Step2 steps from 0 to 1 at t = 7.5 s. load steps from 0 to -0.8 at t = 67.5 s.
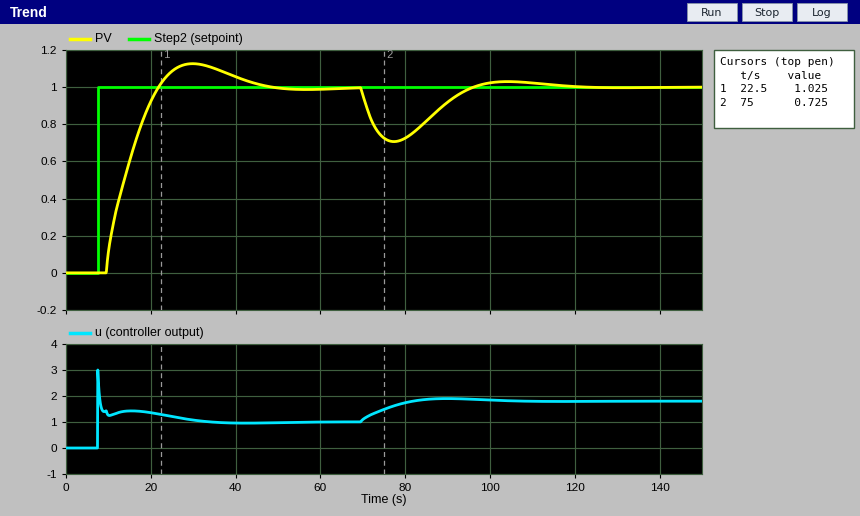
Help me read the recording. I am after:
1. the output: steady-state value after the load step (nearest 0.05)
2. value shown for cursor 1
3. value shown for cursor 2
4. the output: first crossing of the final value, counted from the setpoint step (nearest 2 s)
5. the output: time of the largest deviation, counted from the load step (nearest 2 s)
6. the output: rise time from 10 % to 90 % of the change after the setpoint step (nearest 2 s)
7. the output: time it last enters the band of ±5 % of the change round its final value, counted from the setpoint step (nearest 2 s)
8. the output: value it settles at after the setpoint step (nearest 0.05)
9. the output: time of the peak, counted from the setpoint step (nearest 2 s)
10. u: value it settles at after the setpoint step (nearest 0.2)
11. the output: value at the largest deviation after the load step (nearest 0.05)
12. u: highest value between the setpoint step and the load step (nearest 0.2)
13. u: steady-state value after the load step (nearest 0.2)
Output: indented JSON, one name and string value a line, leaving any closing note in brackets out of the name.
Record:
{
  "the output: steady-state value after the load step": "1.00",
  "value shown for cursor 1": "1.025",
  "value shown for cursor 2": "0.725",
  "the output: first crossing of the final value, counted from the setpoint step": "14 s",
  "the output: time of the largest deviation, counted from the load step": "10 s",
  "the output: rise time from 10 % to 90 % of the change after the setpoint step": "10 s",
  "the output: time it last enters the band of ±5 % of the change round its final value, counted from the setpoint step": "34 s",
  "the output: value it settles at after the setpoint step": "1.00",
  "the output: time of the peak, counted from the setpoint step": "22 s",
  "u: value it settles at after the setpoint step": "1.0",
  "the output: value at the largest deviation after the load step": "0.70",
  "u: highest value between the setpoint step and the load step": "3.0",
  "u: steady-state value after the load step": "1.8"
}
